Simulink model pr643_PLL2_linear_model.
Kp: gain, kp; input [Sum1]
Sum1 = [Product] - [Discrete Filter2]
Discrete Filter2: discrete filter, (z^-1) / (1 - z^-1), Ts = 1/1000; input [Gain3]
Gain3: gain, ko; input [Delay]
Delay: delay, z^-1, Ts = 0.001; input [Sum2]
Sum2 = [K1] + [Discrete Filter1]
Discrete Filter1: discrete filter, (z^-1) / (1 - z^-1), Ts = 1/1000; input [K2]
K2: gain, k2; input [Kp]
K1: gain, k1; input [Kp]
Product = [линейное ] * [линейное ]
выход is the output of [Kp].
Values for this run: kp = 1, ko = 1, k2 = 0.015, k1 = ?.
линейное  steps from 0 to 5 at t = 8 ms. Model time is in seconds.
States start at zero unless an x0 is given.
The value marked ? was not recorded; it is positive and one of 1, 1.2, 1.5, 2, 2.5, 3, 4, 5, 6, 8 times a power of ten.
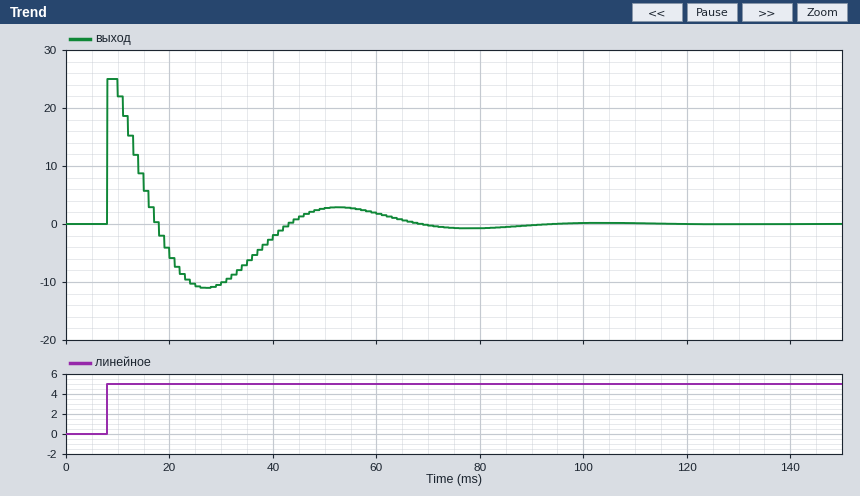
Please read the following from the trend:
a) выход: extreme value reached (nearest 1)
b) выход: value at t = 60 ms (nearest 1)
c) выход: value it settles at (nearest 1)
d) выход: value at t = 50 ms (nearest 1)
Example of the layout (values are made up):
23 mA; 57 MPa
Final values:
25; 2; 0; 3
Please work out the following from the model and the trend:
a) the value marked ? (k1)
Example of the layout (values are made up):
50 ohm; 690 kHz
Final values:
0.12
